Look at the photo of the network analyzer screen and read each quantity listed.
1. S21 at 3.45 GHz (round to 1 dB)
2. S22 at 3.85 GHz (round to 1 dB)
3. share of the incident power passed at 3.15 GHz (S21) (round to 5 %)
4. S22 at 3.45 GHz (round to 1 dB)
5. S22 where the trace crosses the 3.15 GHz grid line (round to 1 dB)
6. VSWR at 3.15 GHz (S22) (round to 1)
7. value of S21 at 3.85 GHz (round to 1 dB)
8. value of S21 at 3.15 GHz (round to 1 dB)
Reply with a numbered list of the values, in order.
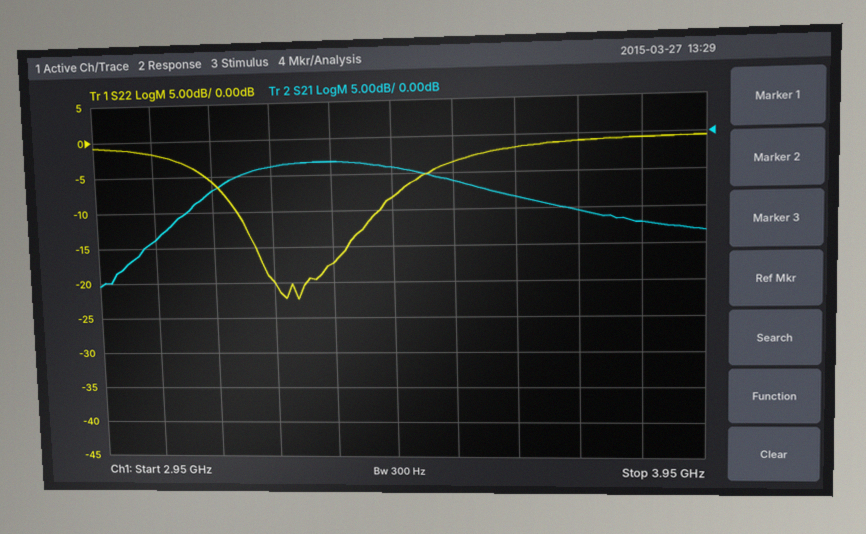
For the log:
1. -4 dB
2. -1 dB
3. 20 %
4. -8 dB
5. -6 dB
6. 3
7. -12 dB
8. -7 dB
